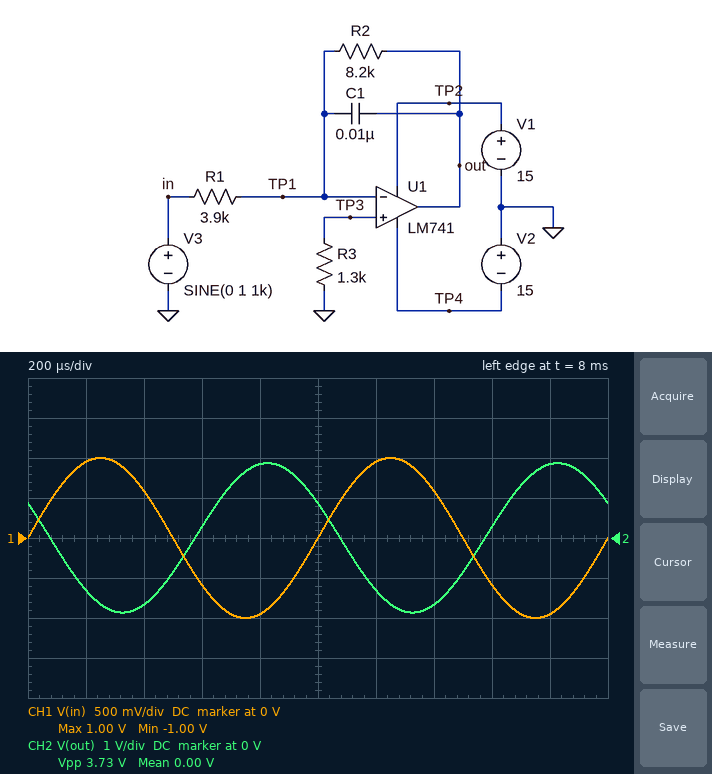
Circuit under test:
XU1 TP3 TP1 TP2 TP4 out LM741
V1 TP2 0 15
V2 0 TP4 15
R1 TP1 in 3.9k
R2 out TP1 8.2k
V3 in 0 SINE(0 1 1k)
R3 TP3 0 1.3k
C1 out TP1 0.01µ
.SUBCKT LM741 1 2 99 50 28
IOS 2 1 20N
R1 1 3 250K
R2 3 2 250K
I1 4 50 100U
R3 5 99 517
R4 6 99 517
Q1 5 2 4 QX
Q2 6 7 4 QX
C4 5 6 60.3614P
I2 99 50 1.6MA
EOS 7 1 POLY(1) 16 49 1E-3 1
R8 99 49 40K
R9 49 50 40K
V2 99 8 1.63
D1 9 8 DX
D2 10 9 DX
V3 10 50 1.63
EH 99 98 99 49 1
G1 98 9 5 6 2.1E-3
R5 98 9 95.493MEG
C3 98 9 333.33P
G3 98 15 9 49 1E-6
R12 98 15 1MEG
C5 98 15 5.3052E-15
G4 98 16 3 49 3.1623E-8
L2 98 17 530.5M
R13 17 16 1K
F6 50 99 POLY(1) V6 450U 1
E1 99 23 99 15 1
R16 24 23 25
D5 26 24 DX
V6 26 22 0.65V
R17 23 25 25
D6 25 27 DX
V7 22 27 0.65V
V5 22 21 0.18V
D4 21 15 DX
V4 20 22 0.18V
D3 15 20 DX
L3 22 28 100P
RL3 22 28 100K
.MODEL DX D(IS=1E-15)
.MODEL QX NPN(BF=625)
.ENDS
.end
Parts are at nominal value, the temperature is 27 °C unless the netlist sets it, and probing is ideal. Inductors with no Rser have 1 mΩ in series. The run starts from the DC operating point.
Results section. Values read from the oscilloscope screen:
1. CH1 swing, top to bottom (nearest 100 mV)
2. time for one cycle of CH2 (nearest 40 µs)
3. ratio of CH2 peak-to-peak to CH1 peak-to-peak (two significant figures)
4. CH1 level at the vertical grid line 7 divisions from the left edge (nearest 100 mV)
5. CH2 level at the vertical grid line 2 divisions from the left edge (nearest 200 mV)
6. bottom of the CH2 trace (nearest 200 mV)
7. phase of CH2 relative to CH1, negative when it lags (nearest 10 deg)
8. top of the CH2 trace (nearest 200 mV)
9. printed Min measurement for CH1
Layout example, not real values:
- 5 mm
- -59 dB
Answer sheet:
- 2.0 V
- 1.00 ms
- 1.9
- 600 mV
- -1.6 V
- -1.8 V
- 150 deg
- 1.8 V
- -1.00 V
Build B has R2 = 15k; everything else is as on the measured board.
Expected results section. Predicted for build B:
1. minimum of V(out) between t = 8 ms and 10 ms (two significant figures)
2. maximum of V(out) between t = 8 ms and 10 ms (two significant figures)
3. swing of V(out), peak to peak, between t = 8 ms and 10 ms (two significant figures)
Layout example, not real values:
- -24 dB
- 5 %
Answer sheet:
- -2.8 V
- 2.8 V
- 5.6 V
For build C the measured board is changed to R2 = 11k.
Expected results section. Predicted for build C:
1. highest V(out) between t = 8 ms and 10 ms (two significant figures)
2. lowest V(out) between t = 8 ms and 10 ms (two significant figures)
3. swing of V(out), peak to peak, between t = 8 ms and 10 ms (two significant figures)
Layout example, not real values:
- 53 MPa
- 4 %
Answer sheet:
- 2.3 V
- -2.3 V
- 4.6 V
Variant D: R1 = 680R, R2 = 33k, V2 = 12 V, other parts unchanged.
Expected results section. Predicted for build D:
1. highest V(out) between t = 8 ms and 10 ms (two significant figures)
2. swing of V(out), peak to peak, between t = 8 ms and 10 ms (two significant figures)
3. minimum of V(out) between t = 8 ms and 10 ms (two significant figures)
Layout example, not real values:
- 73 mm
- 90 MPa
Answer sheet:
- 14 V
- 25 V
- -11 V
